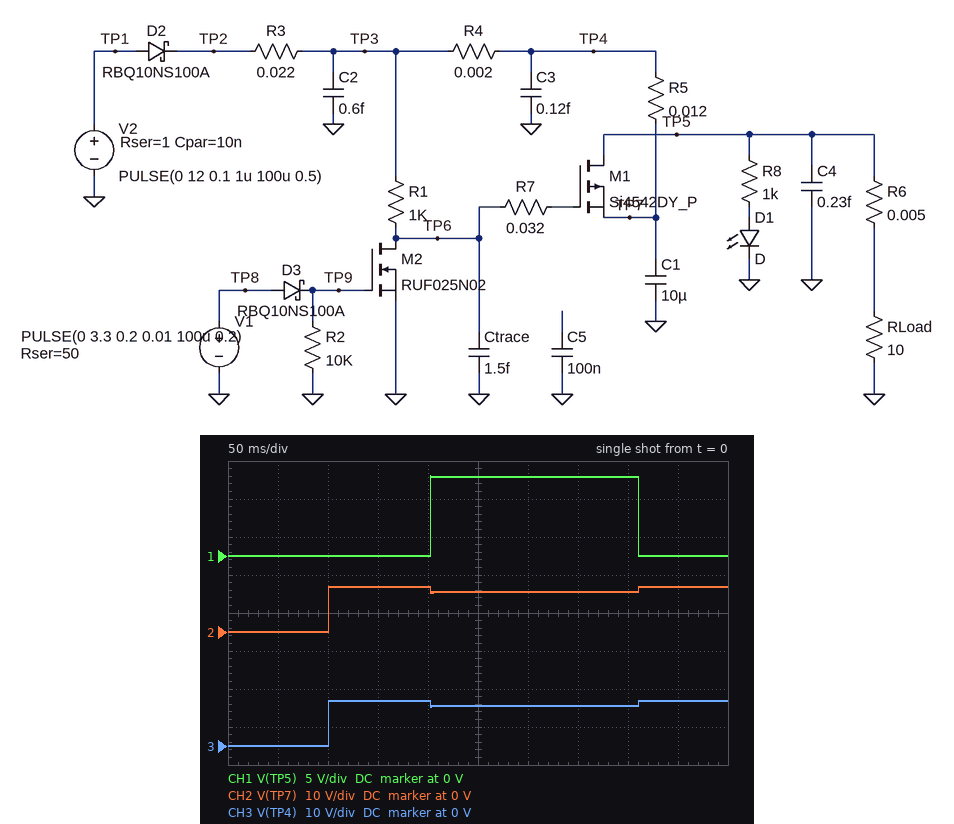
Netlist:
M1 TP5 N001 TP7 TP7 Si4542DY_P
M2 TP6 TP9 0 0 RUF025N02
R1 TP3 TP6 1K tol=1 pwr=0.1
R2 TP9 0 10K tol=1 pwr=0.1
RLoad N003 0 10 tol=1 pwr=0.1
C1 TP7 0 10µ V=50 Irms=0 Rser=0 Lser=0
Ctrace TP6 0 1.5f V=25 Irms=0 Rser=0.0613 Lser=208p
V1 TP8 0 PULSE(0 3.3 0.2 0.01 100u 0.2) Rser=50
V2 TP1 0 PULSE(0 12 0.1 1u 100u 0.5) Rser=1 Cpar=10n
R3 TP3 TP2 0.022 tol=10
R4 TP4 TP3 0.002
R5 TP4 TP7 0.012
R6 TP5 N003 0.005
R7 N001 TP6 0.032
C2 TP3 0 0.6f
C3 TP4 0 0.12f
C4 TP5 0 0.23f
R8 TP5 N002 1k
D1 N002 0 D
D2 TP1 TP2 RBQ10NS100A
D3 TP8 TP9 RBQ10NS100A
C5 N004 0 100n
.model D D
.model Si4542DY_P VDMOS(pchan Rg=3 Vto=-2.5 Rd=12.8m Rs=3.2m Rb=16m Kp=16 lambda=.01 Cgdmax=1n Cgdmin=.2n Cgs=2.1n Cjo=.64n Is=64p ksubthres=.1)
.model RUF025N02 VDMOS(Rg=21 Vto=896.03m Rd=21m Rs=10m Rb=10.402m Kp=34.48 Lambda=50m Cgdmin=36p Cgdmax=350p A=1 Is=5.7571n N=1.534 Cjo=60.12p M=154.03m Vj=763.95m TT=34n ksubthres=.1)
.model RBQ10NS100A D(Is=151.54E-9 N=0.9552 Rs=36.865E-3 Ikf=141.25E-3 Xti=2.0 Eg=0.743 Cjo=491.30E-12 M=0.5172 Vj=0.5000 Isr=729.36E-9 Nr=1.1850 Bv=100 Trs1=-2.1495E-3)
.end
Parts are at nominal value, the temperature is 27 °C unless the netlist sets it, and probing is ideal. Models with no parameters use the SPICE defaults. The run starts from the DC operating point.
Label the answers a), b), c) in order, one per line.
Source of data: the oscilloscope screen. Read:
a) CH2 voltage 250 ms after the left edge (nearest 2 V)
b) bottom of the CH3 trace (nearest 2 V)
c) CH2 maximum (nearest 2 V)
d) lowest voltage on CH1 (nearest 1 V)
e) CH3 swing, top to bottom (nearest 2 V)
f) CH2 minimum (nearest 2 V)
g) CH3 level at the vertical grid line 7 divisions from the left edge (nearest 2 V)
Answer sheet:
a) 10 V
b) 0 V
c) 12 V
d) 0 V
e) 12 V
f) 0 V
g) 10 V
